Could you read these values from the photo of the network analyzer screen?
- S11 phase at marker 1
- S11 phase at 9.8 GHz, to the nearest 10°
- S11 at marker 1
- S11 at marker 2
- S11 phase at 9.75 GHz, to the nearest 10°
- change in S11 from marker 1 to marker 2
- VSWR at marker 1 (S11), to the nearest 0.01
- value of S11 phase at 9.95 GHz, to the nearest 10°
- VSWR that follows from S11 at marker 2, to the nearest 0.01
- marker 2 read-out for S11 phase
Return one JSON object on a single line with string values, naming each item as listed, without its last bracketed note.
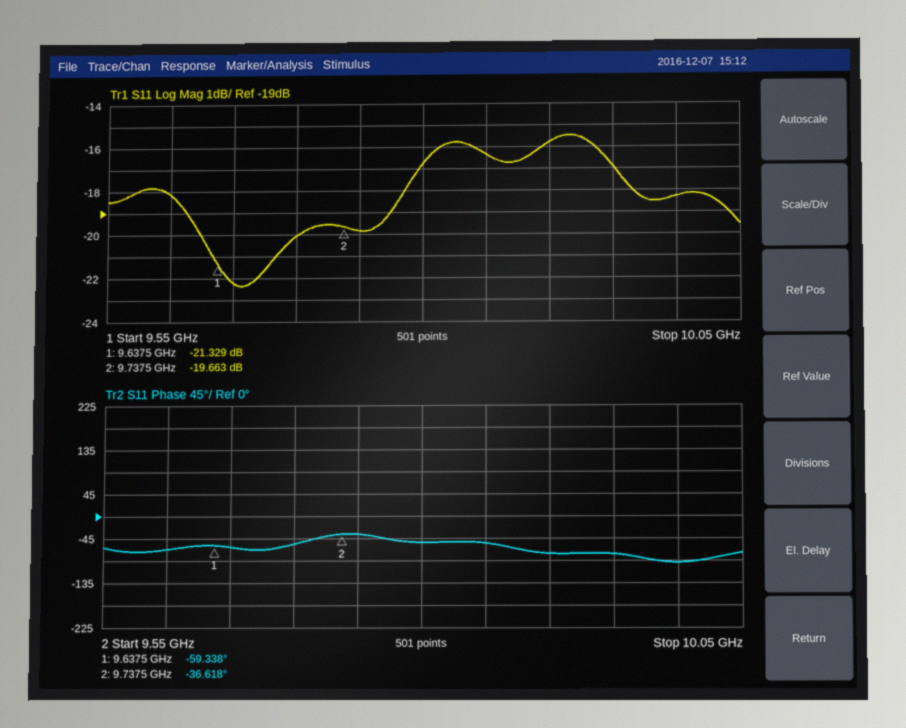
{"S11 phase at marker 1": "-59.338°", "S11 phase at 9.8 GHz, to the nearest 10°": "-50°", "S11 at marker 1": "-21.329 dB", "S11 at marker 2": "-19.663 dB", "S11 phase at 9.75 GHz, to the nearest 10°": "-40°", "change in S11 from marker 1 to marker 2": "1.666 dB", "VSWR at marker 1 (S11), to the nearest 0.01": "1.19", "value of S11 phase at 9.95 GHz, to the nearest 10°": "-80°", "VSWR that follows from S11 at marker 2, to the nearest 0.01": "1.23", "marker 2 read-out for S11 phase": "-36.618°"}
